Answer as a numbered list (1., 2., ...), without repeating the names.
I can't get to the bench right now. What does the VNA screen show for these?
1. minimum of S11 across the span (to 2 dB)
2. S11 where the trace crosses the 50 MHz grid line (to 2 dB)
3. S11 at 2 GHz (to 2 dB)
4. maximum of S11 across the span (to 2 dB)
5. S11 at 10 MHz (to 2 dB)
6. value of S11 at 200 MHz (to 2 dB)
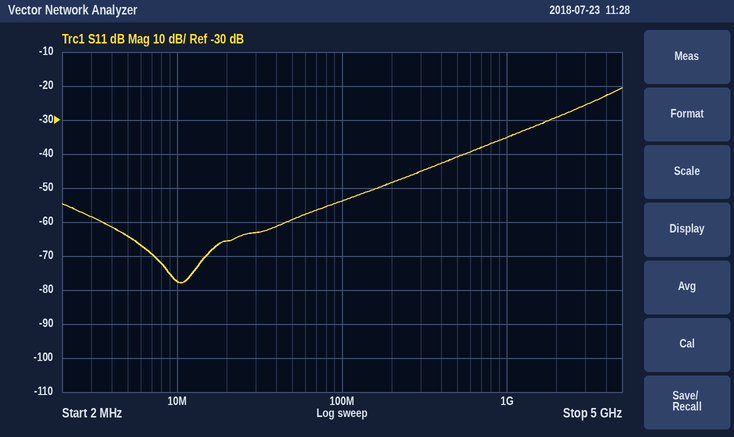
1. -78 dB
2. -60 dB
3. -30 dB
4. -20 dB
5. -78 dB
6. -48 dB
